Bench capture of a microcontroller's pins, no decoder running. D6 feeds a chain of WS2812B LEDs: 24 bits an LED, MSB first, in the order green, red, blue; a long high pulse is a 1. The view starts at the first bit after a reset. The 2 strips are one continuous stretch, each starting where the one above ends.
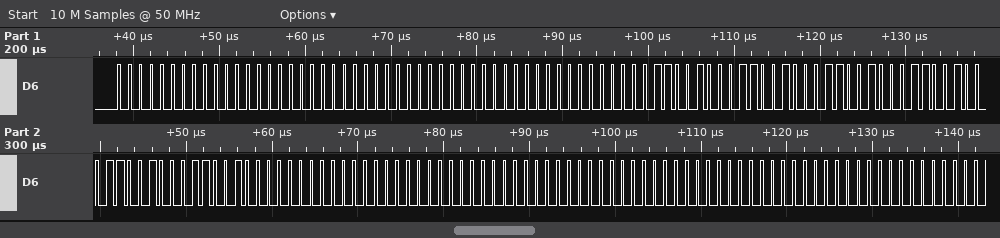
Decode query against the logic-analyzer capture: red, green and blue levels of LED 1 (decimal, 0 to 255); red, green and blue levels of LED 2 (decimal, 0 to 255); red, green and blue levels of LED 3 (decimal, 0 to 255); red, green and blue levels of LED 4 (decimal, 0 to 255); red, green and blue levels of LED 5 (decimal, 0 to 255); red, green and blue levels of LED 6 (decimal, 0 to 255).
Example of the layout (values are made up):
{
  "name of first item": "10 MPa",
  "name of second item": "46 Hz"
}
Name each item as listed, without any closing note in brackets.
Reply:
{
  "red, green and blue levels of LED 1": "0, 0, 0",
  "red, green and blue levels of LED 2": "0, 0, 0",
  "red, green and blue levels of LED 3": "50, 50, 50",
  "red, green and blue levels of LED 4": "50, 50, 50",
  "red, green and blue levels of LED 5": "0, 0, 0",
  "red, green and blue levels of LED 6": "0, 0, 0"
}
